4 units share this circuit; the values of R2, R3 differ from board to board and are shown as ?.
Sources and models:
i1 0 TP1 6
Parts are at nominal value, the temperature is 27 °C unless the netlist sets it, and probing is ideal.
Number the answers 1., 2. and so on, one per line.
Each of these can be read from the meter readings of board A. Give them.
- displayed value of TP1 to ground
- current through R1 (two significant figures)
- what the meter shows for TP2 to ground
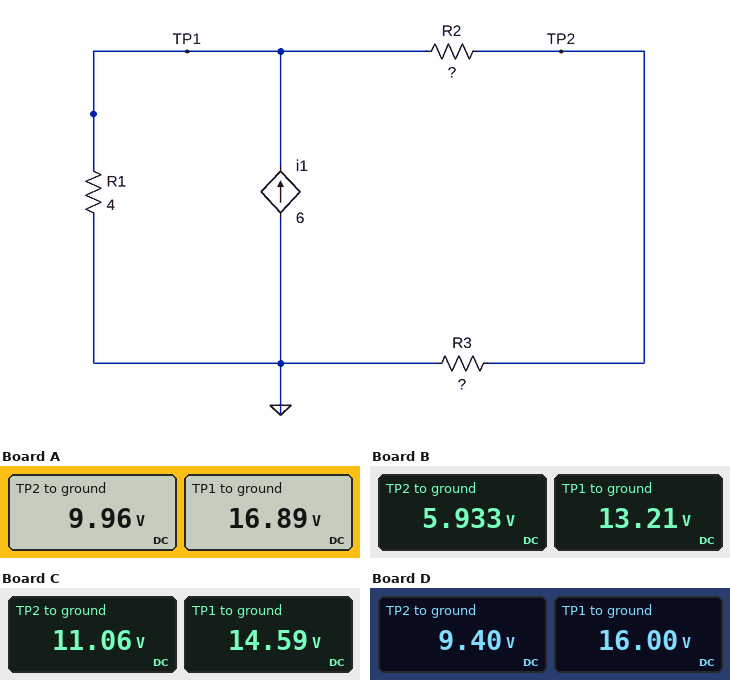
1. 16.89 V
2. 4.2 A
3. 9.96 V
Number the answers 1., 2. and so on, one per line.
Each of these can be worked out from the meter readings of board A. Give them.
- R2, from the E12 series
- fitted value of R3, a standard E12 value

1. 3.9 Ω
2. 5.6 Ω
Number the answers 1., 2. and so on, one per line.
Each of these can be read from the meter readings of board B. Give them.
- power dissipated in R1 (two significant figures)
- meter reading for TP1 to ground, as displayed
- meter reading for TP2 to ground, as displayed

1. 44 W
2. 13.21 V
3. 5.933 V
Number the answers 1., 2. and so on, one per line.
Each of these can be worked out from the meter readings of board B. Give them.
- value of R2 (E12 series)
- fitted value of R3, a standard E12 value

1. 2.7 Ω
2. 2.2 Ω
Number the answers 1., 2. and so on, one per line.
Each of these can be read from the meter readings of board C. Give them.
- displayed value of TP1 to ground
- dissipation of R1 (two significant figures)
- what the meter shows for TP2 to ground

1. 14.59 V
2. 53 W
3. 11.06 V
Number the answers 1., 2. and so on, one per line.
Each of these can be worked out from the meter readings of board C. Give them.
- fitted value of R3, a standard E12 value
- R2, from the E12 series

1. 4.7 Ω
2. 1.5 Ω
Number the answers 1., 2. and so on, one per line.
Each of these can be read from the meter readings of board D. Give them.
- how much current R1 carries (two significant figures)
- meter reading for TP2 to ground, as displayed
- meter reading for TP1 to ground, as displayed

1. 4.0 A
2. 9.40 V
3. 16.00 V
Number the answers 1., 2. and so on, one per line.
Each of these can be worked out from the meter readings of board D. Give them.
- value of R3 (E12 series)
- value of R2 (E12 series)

1. 4.7 Ω
2. 3.3 Ω
